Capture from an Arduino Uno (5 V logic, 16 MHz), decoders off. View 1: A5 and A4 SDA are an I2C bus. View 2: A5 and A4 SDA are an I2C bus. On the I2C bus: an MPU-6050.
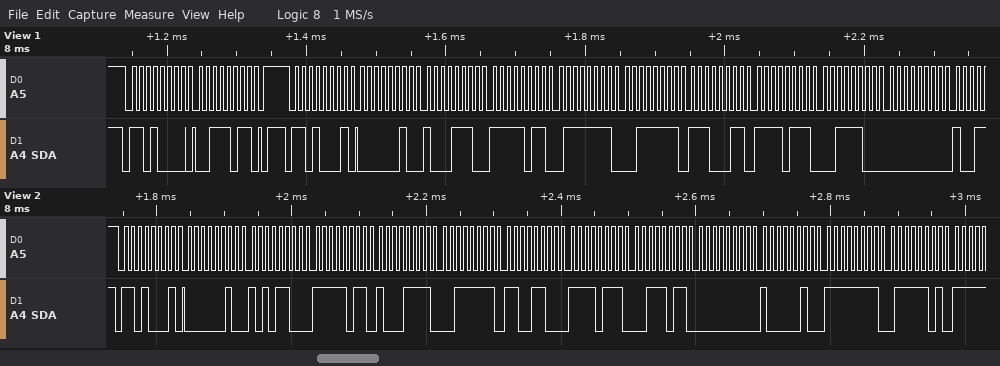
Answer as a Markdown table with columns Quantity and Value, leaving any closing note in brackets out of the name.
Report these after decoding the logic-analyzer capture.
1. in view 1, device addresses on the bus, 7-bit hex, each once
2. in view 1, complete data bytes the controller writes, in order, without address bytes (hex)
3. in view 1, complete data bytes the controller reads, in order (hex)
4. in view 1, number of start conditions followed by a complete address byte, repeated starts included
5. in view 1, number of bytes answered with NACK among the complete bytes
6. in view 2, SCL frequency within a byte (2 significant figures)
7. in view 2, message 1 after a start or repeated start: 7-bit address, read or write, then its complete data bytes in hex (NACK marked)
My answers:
| Quantity | Value |
|---|---|
| in view 1, device addresses on the bus, 7-bit hex, each once | 0x68 |
| in view 1, complete data bytes the controller writes, in order, without address bytes | 3B |
| in view 1, complete data bytes the controller reads, in order | 02 8E FB 7F 3F E3 F7 3C 00 |
| in view 1, number of start conditions followed by a complete address byte, repeated starts included | 2 |
| in view 1, number of bytes answered with NACK among the complete bytes | 0 |
| in view 2, SCL frequency within a byte | 100 kHz |
| in view 2, message 1 after a start or repeated start: 7-bit address, read or write, then its complete data bytes in hex | 0x68 read: 02 AC FB 8F 3F CC F7 3B 00 82 FF 7D |
